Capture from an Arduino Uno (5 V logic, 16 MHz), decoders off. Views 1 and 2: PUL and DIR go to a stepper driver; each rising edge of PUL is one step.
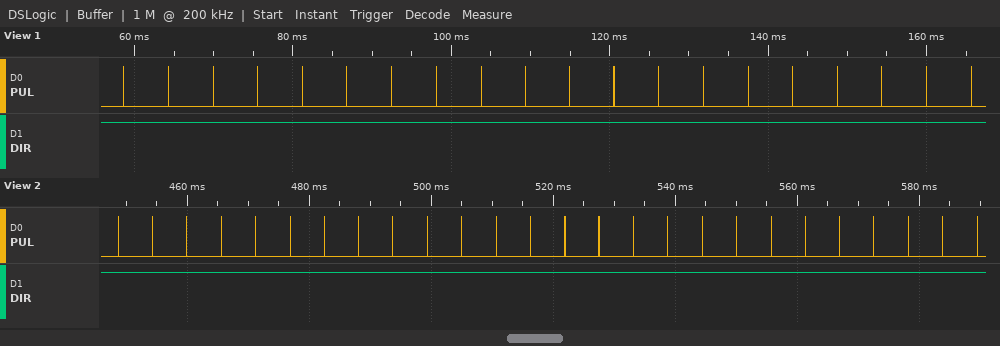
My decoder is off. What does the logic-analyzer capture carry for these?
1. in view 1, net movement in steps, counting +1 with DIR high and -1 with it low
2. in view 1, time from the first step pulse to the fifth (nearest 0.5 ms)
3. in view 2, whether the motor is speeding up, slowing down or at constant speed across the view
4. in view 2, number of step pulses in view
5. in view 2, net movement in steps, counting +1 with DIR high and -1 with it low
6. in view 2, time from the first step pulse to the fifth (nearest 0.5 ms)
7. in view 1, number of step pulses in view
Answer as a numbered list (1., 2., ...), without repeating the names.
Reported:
1. +20
2. 22.5 ms
3. constant speed
4. 26
5. +26
6. 22.5 ms
7. 20
